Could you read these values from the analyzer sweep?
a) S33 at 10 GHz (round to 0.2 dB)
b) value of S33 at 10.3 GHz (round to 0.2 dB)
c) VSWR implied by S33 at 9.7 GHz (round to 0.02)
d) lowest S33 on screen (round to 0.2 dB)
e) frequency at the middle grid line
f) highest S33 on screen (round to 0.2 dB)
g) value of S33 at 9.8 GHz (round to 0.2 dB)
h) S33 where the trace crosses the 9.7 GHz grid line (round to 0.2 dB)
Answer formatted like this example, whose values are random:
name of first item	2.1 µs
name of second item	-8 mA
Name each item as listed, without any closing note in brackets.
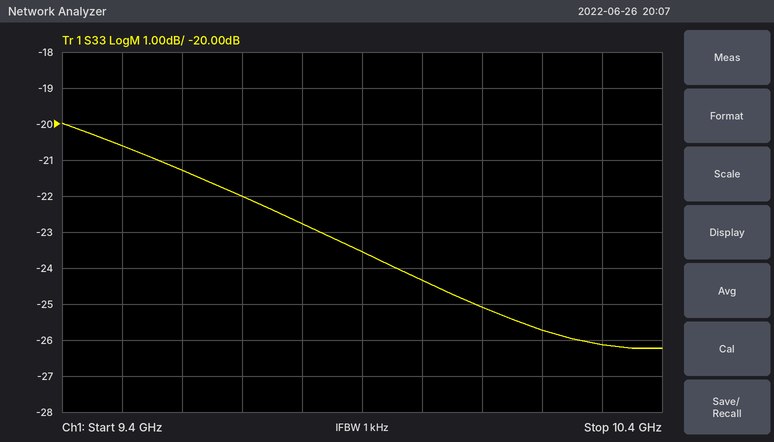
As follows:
S33 at 10 GHz	-24.4 dB
value of S33 at 10.3 GHz	-26.2 dB
VSWR implied by S33 at 9.7 GHz	1.18
lowest S33 on screen	-26.2 dB
frequency at the middle grid line	9.9 GHz
highest S33 on screen	-20.0 dB
value of S33 at 9.8 GHz	-22.8 dB
S33 where the trace crosses the 9.7 GHz grid line	-22.0 dB
